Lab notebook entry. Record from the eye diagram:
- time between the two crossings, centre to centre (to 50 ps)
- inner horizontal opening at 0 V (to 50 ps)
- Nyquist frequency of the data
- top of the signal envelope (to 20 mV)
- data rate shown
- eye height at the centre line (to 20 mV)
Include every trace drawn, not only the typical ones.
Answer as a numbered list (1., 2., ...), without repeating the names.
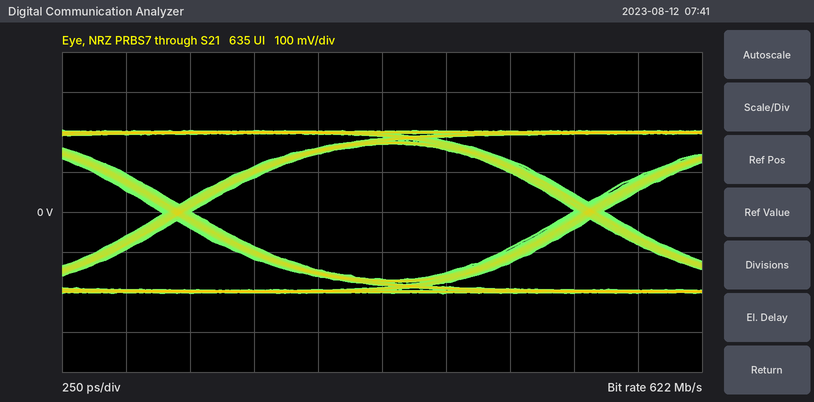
1. 1.60 ns
2. 1.50 ns
3. 311 MHz
4. 200 mV
5. 622 Mb/s
6. 340 mV
